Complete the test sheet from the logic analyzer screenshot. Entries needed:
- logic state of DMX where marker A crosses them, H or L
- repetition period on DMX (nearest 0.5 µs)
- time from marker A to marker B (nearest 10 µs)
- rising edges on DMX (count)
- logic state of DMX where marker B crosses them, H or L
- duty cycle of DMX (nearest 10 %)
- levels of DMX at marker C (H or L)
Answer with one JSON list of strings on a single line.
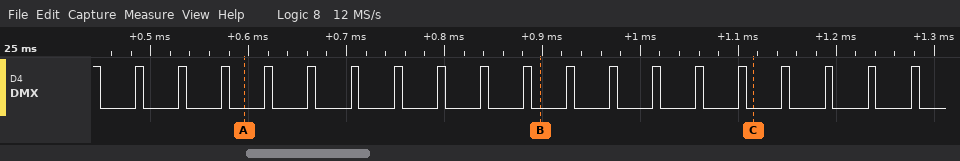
["DMX=L", "44 µs", "300 µs", "19", "DMX=L", "20 %", "DMX=L"]
